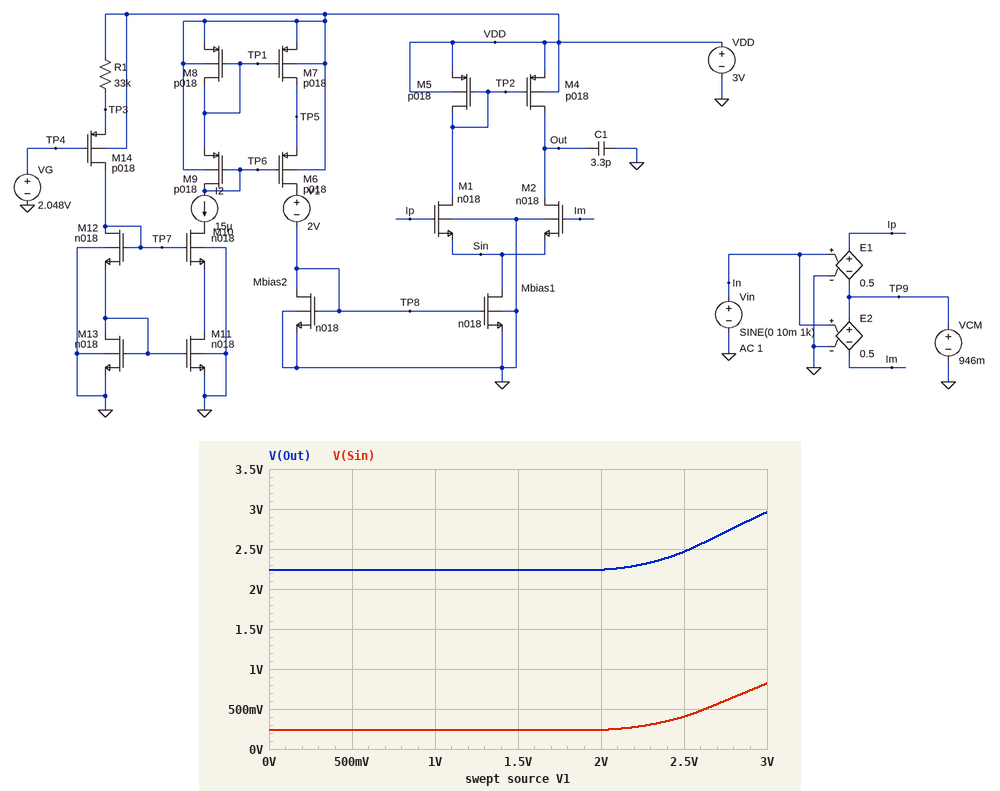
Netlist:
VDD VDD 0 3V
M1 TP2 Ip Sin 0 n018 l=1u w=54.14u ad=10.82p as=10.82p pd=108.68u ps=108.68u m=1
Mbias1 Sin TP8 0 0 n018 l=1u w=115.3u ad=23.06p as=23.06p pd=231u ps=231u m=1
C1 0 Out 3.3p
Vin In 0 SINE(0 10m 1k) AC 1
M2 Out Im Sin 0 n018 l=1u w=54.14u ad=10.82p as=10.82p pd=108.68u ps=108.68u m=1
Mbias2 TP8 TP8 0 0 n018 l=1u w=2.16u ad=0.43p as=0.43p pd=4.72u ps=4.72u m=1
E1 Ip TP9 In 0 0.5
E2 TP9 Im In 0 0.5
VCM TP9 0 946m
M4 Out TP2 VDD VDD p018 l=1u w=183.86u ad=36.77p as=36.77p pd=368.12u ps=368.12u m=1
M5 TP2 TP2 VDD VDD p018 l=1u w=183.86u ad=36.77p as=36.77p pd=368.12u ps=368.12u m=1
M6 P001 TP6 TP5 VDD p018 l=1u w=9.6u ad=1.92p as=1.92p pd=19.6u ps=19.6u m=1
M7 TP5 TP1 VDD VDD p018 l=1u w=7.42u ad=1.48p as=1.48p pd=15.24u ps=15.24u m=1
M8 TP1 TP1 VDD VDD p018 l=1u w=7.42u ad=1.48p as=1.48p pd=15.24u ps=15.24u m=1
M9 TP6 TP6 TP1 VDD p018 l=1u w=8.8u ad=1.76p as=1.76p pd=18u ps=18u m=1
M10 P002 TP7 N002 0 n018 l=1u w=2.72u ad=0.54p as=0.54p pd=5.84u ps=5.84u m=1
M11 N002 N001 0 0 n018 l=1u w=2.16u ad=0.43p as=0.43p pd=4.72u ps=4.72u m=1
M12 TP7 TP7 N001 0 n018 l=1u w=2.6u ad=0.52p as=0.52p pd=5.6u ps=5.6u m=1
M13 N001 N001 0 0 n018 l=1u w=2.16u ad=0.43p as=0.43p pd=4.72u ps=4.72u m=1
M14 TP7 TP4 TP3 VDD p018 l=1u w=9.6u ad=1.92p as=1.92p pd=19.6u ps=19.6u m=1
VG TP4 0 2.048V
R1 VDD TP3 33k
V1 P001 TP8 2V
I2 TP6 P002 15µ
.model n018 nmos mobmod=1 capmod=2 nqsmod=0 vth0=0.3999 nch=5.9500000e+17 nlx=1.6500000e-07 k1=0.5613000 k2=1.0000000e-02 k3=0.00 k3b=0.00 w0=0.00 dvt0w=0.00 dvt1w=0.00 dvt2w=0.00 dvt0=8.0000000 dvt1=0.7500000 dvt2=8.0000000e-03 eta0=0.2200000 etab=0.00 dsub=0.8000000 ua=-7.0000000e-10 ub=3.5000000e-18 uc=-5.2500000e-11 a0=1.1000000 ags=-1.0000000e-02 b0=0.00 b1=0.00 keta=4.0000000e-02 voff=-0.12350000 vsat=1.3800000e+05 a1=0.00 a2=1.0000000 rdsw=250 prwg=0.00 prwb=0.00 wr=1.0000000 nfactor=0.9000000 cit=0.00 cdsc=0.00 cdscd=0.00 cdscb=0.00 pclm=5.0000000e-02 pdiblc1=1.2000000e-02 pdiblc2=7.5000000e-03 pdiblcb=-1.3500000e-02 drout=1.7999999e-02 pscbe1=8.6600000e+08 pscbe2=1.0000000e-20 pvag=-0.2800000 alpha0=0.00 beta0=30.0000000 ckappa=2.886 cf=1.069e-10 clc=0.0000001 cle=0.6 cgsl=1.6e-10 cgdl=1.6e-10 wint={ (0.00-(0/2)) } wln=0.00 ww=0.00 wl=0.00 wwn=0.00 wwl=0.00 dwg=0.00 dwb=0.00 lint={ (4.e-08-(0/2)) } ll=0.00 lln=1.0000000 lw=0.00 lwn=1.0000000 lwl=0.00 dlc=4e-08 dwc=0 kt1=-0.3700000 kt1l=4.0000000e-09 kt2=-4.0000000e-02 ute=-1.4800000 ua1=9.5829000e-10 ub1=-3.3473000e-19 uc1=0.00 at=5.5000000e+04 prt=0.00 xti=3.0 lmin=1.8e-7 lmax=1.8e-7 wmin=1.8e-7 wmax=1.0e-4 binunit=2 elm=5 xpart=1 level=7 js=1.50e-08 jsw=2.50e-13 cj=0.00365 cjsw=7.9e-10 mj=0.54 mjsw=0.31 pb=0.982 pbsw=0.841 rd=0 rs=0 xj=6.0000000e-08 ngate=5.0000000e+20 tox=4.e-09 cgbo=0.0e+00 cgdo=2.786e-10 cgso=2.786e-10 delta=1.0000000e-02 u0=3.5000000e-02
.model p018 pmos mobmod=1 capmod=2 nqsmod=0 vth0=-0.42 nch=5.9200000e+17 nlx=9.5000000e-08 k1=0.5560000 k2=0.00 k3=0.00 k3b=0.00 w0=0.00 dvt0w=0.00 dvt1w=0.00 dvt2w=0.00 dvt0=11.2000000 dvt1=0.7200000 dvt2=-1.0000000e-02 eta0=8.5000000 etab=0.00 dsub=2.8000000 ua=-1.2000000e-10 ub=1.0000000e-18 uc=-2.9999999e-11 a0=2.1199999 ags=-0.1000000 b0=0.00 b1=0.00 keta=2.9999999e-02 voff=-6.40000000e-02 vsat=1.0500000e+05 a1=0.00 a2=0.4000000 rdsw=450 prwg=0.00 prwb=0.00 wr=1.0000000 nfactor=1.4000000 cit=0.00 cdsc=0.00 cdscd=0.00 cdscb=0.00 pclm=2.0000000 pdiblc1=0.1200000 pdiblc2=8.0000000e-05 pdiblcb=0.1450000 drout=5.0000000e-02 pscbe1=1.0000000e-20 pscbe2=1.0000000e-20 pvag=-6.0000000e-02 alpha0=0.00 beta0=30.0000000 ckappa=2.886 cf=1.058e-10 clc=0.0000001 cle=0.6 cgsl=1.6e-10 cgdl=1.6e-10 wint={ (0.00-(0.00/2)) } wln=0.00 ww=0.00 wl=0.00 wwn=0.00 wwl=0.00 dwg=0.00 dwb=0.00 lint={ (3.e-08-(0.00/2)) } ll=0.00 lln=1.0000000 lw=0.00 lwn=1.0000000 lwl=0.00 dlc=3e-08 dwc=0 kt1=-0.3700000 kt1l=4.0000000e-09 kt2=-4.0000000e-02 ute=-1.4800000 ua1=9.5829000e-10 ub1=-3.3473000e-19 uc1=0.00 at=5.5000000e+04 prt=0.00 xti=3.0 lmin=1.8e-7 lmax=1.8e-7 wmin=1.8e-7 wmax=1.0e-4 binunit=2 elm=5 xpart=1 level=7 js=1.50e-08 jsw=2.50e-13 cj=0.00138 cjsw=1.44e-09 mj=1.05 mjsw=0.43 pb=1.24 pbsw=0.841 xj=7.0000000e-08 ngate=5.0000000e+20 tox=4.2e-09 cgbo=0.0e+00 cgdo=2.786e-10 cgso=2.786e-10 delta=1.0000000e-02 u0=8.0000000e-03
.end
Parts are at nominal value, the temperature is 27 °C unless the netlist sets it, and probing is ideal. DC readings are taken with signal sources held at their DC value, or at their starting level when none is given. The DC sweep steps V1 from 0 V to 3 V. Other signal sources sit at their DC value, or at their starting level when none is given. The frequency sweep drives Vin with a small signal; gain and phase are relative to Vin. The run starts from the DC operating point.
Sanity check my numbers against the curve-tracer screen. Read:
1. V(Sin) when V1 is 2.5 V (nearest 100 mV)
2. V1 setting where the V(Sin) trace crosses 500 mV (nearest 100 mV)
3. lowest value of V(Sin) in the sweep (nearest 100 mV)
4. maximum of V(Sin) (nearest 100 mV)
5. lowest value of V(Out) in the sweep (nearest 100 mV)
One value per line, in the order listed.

400 mV
2.6 V
200 mV
800 mV
2.2 V
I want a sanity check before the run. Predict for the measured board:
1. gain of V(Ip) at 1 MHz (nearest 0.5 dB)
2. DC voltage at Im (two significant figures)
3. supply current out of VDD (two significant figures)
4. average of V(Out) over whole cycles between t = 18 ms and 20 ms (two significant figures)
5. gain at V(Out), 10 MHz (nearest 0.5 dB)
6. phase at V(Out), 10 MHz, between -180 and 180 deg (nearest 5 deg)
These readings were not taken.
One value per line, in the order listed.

-6.0 dB
950 mV
1.0 mA
2.2 V
20.0 dB
-75 deg
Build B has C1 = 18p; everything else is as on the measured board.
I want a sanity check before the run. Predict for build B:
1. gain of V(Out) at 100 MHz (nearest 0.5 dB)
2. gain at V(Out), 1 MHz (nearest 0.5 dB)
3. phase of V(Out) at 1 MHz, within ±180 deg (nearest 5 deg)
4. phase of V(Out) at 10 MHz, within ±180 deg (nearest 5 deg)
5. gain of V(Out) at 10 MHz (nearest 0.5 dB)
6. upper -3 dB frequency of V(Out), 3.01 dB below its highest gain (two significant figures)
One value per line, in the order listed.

-14.5 dB
25.5 dB
-60 deg
-90 deg
6.5 dB
630 kHz
